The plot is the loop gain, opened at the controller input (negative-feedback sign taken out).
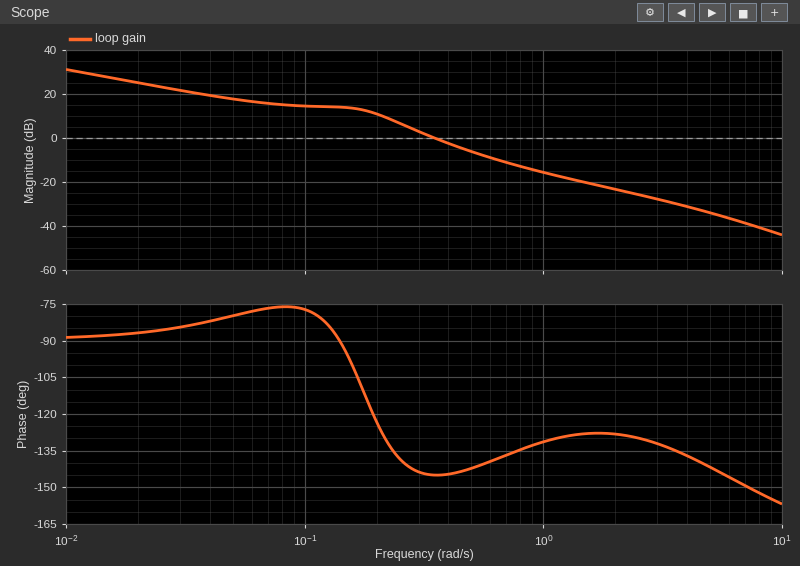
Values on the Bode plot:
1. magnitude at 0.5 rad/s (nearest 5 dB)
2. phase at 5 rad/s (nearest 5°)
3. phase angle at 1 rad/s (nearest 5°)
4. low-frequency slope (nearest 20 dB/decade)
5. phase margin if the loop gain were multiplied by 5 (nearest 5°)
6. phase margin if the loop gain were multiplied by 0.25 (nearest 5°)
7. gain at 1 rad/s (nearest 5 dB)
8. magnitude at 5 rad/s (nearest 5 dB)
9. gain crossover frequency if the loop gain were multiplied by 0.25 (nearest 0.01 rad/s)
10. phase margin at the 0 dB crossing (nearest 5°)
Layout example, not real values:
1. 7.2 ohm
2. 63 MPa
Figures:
1. -5 dB
2. -140°
3. -130°
4. -20 dB/decade
5. 45°
6. 65°
7. -15 dB
8. -35 dB
9. 0.19 rad/s
10. 35°
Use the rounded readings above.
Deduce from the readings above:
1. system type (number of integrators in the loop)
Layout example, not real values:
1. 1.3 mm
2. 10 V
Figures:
1. 1
